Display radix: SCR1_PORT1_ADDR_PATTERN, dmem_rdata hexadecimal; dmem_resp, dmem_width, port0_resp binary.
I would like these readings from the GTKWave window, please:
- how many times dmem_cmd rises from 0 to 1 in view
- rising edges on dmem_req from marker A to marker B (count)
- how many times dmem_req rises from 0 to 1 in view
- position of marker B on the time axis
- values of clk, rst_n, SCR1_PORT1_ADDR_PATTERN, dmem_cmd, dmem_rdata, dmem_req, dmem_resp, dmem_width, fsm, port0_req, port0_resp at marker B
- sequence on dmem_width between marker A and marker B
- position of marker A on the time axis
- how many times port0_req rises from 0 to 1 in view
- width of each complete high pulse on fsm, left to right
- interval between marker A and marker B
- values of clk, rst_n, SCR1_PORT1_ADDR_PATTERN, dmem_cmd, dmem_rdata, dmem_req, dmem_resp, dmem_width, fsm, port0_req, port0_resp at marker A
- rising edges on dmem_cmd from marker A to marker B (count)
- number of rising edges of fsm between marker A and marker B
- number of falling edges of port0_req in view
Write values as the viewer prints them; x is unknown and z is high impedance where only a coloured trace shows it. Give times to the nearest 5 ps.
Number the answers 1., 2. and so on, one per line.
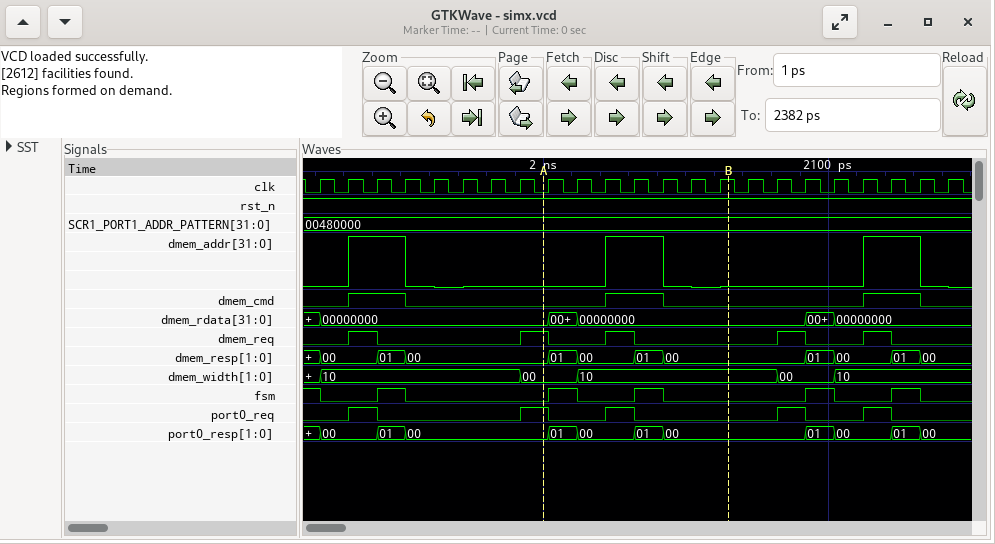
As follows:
1. 3
2. 1
3. 5
4. 2065 ps
5. clk=1, rst_n=1, SCR1_PORT1_ADDR_PATTERN=00480000, dmem_cmd=0, dmem_rdata=00000000, dmem_req=0, dmem_resp=00, dmem_width=10, fsm=0, port0_req=0, port0_resp=00
6. 00, 10
7. 2000 ps
8. 5
9. 10 ps, 10 ps, 10 ps, 10 ps, 10 ps
10. 65 ps
11. clk=0, rst_n=1, SCR1_PORT1_ADDR_PATTERN=00480000, dmem_cmd=0, dmem_rdata=00000000, dmem_req=1, dmem_resp=00, dmem_width=00, fsm=0, port0_req=1, port0_resp=00
12. 1
13. 2
14. 5
